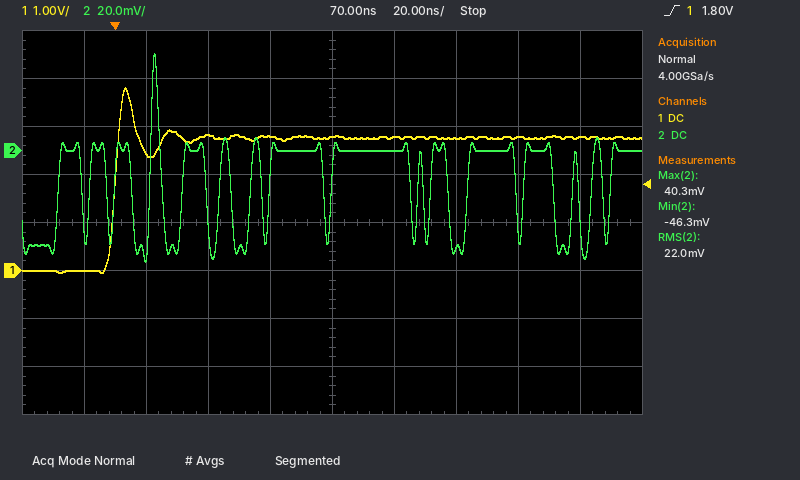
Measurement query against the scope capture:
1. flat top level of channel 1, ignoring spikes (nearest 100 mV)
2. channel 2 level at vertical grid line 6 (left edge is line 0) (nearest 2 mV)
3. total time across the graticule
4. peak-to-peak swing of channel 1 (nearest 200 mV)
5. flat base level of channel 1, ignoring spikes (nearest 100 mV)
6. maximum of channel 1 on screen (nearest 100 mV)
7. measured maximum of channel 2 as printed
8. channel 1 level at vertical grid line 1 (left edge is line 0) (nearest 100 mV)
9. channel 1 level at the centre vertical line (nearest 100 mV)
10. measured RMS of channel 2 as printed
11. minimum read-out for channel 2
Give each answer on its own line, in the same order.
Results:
2.8 V
0 mV
200 ns
3.8 V
0.0 V
3.8 V
40.3 mV
0.0 V
2.8 V
22.0 mV
-46.3 mV
